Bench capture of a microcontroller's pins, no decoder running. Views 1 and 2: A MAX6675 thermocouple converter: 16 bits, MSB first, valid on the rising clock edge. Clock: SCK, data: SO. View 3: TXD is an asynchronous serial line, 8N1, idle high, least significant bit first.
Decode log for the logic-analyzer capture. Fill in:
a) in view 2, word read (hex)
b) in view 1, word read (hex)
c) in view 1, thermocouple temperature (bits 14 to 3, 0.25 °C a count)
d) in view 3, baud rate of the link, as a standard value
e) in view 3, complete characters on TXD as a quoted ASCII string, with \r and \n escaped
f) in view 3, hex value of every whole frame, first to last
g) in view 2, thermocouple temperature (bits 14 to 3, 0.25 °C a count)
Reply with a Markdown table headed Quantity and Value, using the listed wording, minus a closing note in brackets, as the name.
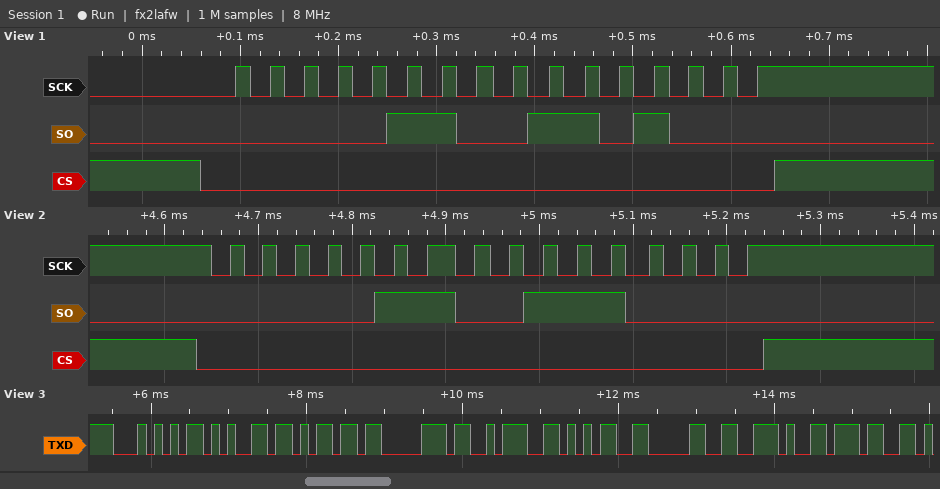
| Quantity | Value |
|---|---|
| in view 2, word read | 0x0670 |
| in view 1, word read | 0x0668 |
| in view 1, thermocouple temperature | 51.25 °C |
| in view 3, baud rate of the link, as a standard value | 9600 baud |
| in view 3, complete characters on TXD as a quoted ASCII string, with \r and \n escaped | "Temp:50.7" |
| in view 3, hex value of every whole frame, first to last | 0x54 0x65 0x6D 0x70 0x3A 0x35 0x30 0x2E 0x37 |
| in view 2, thermocouple temperature | 51.50 °C |
